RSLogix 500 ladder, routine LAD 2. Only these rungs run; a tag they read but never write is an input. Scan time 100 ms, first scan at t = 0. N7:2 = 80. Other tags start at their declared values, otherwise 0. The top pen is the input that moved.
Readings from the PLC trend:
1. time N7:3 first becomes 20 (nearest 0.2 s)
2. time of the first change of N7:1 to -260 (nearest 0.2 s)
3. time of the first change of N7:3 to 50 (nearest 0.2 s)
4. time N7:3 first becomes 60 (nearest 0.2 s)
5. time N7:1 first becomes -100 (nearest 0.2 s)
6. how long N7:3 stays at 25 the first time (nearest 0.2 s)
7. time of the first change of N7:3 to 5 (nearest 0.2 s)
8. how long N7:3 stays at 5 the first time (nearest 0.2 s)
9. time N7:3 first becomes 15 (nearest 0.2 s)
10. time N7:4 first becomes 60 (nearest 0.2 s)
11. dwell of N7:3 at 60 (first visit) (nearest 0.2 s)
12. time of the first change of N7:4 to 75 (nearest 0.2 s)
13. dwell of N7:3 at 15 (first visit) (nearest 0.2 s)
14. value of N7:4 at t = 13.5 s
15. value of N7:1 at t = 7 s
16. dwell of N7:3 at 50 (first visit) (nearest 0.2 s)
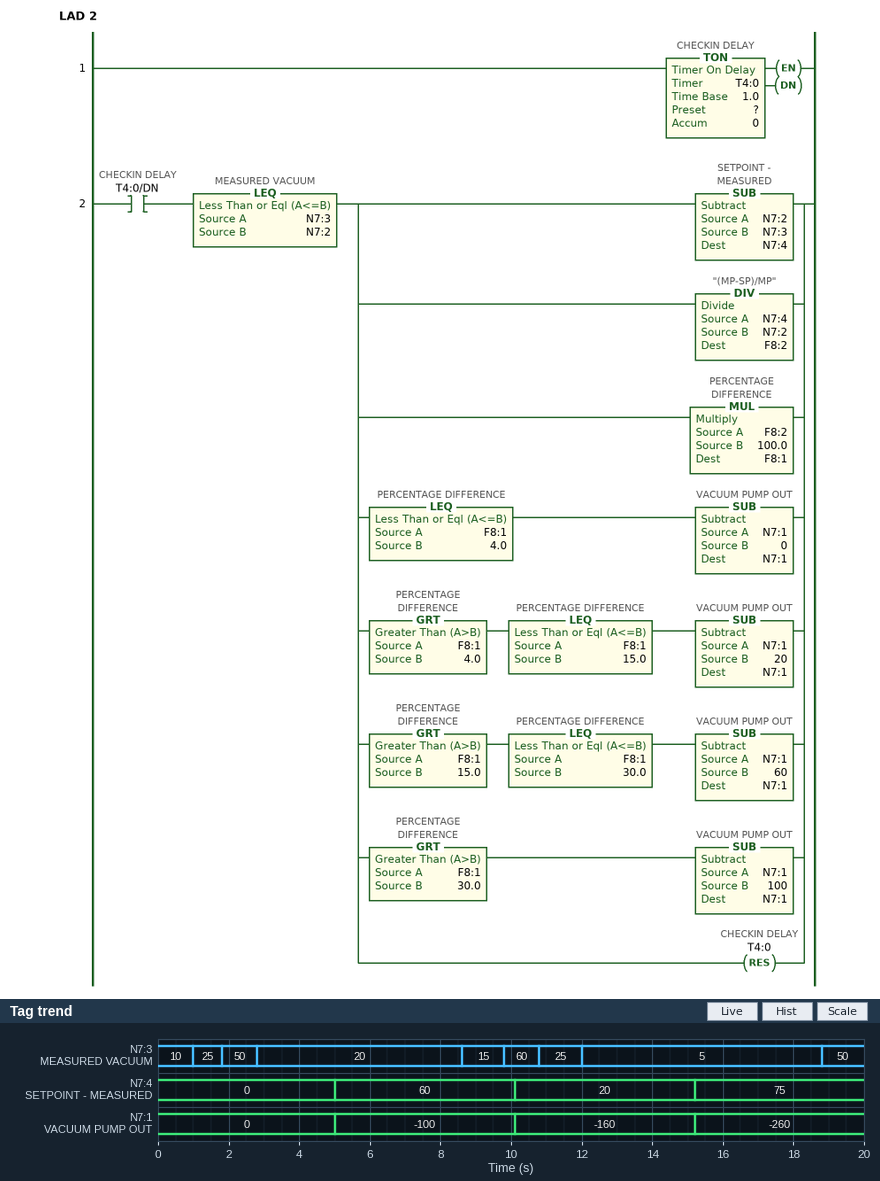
2.8 s
15.2 s
1.8 s
9.8 s
5.0 s
0.8 s
12.0 s
6.8 s
8.6 s
5.0 s
1.0 s
15.2 s
1.2 s
20
-100
1.0 s
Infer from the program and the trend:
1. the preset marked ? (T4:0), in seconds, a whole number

5 s
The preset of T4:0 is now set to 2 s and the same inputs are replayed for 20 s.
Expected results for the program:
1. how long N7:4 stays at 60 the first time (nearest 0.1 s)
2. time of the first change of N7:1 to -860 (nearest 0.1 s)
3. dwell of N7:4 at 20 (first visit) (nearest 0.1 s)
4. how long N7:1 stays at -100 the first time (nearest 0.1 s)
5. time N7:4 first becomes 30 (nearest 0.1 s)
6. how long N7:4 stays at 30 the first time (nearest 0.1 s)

6.3 s
18.8 s
2.1 s
2.1 s
2.0 s
2.1 s
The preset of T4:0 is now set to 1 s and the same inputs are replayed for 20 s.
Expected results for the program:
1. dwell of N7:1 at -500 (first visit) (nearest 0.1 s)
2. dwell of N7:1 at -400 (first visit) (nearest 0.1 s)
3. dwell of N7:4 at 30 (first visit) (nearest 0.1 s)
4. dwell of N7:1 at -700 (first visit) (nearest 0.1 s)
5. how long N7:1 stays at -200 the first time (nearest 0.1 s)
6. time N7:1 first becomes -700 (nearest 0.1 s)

1.1 s
1.1 s
1.1 s
1.1 s
1.1 s
7.6 s
